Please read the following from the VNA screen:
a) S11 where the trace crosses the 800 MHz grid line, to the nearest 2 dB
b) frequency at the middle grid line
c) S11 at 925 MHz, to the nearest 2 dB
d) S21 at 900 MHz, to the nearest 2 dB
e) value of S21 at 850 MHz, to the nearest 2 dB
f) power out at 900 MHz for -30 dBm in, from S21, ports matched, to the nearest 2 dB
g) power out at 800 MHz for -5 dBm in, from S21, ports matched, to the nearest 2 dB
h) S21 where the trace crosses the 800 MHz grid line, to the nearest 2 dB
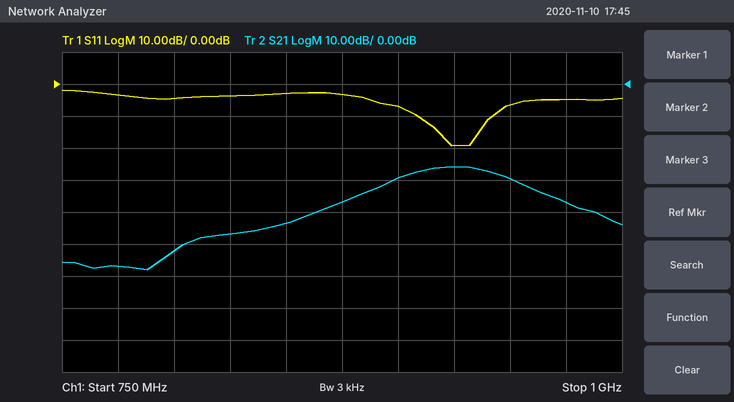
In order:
-4 dB
875 MHz
-20 dB
-30 dB
-44 dB
-60 dBm
-58 dBm
-52 dB
